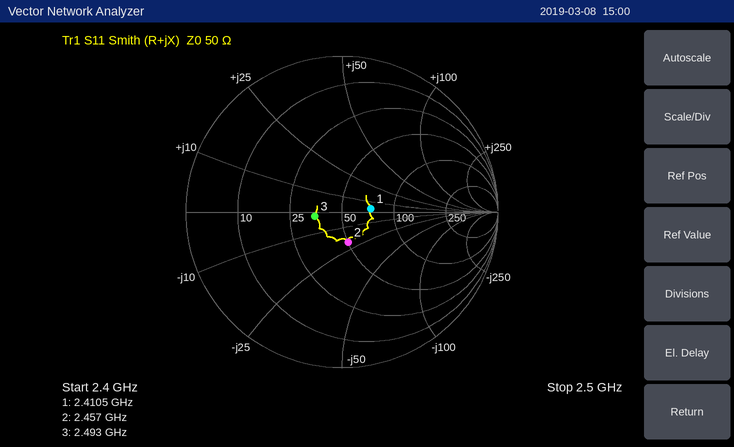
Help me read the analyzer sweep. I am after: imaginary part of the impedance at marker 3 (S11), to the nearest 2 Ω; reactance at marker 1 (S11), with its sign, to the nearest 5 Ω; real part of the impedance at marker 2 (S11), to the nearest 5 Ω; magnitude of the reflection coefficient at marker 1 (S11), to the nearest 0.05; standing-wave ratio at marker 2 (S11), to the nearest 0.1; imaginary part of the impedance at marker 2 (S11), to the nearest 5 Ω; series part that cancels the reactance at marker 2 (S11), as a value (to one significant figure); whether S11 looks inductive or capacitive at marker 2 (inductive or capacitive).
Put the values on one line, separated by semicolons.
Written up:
-2 Ω; +5 Ω; 50 Ω; 0.20; 1.5; -20 Ω; 1 nH; capacitive
